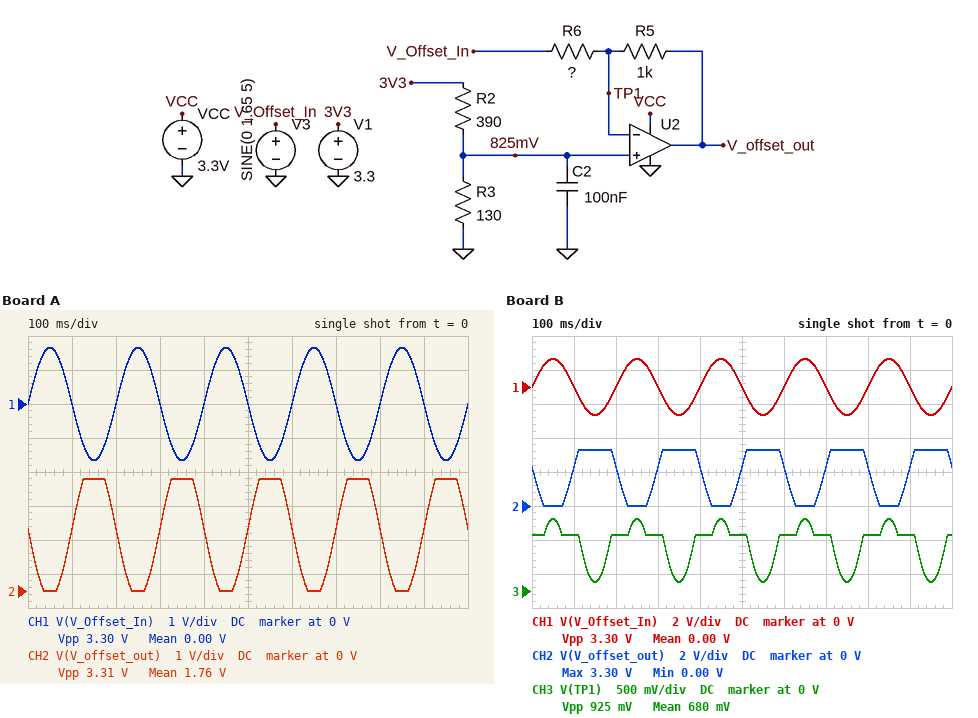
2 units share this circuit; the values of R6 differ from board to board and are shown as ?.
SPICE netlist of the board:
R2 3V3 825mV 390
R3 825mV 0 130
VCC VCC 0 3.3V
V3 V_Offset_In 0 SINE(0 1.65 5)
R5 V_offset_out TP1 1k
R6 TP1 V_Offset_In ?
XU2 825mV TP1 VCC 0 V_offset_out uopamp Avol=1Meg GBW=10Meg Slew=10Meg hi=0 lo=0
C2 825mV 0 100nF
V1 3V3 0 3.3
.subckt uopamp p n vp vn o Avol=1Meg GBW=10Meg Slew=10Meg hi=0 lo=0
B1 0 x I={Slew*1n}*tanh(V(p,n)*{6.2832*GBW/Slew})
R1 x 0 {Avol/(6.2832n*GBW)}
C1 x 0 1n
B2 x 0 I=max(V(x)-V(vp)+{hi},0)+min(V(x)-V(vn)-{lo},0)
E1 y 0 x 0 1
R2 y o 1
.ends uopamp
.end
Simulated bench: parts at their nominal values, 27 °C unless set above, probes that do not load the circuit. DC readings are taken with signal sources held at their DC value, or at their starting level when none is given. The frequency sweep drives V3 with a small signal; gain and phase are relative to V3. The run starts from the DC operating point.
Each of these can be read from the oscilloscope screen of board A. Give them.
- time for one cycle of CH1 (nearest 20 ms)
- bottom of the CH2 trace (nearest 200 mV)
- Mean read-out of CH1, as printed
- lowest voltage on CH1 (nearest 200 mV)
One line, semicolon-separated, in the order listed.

200 ms; 0 V; 0.00 V; -1.6 V
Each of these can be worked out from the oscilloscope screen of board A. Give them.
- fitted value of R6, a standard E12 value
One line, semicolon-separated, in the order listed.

820 Ω
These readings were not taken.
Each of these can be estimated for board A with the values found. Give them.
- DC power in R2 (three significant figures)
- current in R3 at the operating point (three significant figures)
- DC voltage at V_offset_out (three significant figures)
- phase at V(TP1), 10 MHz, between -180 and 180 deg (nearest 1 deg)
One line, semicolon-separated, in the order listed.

15.7 mW; 6.35 mA; 1.83 V; 24 deg
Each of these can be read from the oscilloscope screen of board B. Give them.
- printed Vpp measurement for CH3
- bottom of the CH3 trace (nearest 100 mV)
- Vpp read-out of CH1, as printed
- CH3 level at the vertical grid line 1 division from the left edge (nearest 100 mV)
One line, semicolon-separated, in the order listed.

925 mV; 100 mV; 3.30 V; 800 mV
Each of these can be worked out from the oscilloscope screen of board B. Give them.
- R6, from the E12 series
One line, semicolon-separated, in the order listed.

560 Ω
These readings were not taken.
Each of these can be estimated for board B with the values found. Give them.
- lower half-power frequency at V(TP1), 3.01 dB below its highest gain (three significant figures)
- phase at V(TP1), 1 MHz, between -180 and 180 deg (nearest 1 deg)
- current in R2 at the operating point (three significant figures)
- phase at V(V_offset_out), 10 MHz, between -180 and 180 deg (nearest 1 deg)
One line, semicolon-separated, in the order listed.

3.59 MHz; 74 deg; 6.35 mA; 110 deg
